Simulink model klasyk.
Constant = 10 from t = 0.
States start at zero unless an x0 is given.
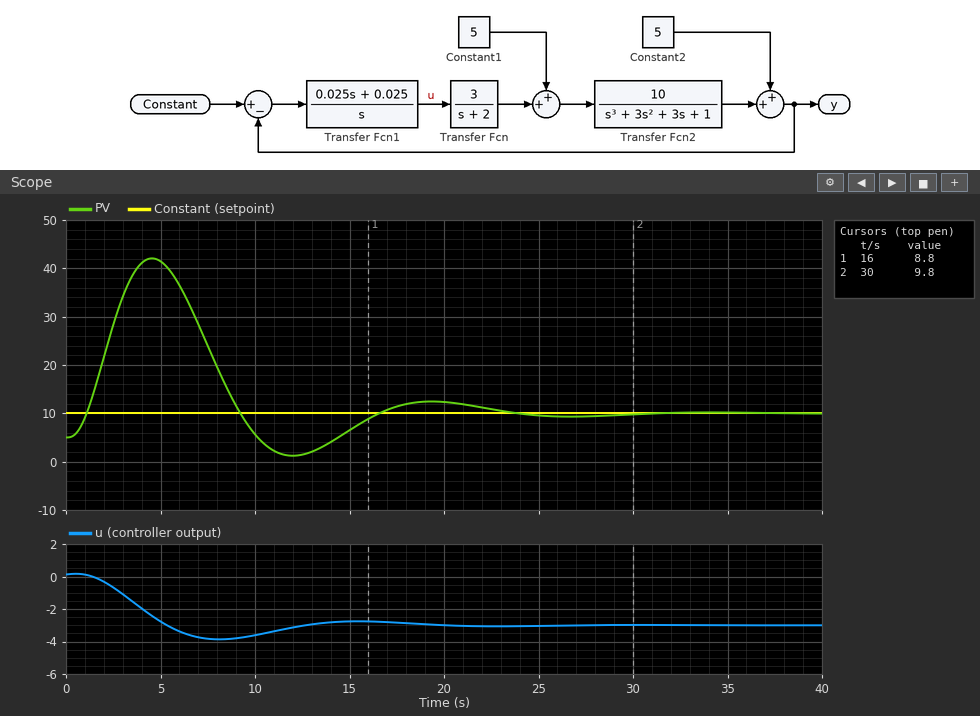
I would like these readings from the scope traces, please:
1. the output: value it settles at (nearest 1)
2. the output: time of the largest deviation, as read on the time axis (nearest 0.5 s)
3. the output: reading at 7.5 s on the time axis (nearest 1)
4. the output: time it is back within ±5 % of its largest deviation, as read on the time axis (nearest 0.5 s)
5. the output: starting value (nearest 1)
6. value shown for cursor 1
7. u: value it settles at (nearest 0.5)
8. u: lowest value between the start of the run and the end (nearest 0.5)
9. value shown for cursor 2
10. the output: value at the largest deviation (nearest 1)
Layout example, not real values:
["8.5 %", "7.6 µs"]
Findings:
["10", "4.5 s", "24", "21.0 s", "5", "8.8", "-3.0", "-4.0", "9.8", "42"]
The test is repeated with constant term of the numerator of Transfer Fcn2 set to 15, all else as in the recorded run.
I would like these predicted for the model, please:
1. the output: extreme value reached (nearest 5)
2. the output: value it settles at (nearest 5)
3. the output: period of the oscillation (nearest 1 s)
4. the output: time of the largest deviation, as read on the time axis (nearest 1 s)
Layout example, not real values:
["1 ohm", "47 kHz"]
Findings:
["55", "10", "12 s", "4 s"]
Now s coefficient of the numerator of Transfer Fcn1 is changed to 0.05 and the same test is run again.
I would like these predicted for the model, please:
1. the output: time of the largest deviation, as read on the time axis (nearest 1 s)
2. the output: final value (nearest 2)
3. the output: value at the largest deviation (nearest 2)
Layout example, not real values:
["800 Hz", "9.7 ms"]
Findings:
["4 s", "10", "40"]
